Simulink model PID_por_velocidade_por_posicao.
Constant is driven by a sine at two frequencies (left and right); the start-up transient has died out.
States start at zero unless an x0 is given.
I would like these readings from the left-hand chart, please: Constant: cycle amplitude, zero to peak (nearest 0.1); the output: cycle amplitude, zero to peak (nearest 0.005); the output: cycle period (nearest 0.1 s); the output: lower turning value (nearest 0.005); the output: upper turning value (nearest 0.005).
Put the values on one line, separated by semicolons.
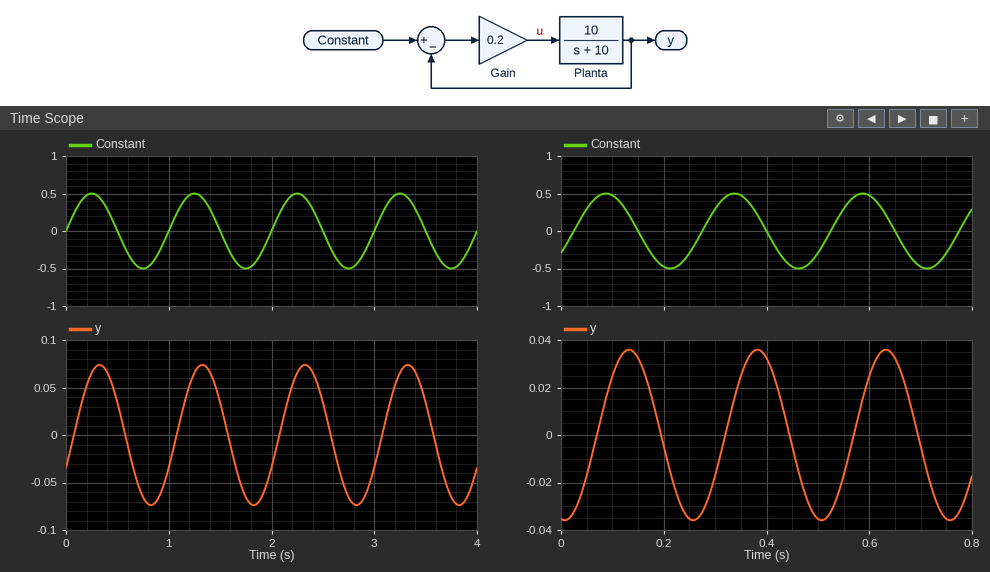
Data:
0.5; 0.075; 1.0 s; -0.075; 0.075
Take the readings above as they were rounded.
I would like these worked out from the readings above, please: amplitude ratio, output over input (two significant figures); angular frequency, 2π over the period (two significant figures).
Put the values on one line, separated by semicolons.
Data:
0.15; 6.3 rad/s
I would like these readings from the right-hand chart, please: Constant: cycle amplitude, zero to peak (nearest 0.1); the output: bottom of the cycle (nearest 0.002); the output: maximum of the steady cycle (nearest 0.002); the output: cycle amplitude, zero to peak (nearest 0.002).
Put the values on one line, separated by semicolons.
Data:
0.5; -0.036; 0.036; 0.036
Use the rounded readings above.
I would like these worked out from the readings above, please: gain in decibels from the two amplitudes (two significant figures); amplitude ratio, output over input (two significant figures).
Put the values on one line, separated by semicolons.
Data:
-23 dB; 0.072
